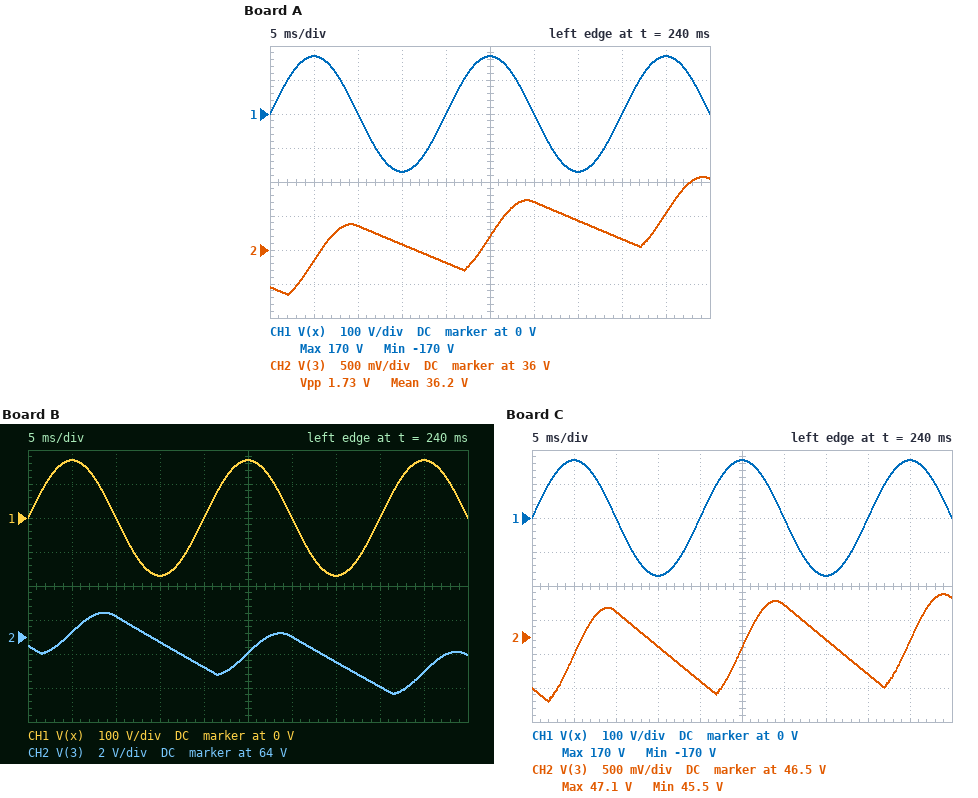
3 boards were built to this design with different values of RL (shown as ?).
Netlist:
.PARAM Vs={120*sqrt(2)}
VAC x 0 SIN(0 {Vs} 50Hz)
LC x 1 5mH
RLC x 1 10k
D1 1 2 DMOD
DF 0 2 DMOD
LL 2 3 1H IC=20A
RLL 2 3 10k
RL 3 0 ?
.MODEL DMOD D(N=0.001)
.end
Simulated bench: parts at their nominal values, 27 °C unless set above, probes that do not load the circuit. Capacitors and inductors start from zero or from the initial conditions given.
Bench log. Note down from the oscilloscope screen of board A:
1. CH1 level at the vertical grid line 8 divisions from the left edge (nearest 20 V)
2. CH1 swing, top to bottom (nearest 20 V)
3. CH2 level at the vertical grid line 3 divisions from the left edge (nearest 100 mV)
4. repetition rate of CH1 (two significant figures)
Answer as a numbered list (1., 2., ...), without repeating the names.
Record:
1. 0 V
2. 340 V
3. 36.1 V
4. 50 Hz
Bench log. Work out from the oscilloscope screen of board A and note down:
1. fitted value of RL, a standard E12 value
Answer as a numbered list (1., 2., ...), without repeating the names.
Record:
1. 1.5 Ω
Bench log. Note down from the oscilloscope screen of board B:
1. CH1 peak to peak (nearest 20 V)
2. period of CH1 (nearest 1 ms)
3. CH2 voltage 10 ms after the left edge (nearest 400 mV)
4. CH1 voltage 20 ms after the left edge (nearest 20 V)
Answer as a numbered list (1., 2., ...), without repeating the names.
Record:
1. 340 V
2. 20 ms
3. 65.2 V
4. 0 V
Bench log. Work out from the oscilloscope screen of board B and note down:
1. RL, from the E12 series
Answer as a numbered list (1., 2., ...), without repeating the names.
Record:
1. 4.7 Ω
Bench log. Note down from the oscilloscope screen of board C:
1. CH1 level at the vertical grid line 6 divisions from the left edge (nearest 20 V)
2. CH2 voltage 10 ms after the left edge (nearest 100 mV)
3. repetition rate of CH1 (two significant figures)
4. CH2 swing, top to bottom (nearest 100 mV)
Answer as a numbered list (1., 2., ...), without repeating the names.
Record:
1. 0 V
2. 46.9 V
3. 50 Hz
4. 1.6 V
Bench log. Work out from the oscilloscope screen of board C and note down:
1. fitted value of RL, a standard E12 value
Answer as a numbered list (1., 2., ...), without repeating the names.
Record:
1. 2.2 Ω
